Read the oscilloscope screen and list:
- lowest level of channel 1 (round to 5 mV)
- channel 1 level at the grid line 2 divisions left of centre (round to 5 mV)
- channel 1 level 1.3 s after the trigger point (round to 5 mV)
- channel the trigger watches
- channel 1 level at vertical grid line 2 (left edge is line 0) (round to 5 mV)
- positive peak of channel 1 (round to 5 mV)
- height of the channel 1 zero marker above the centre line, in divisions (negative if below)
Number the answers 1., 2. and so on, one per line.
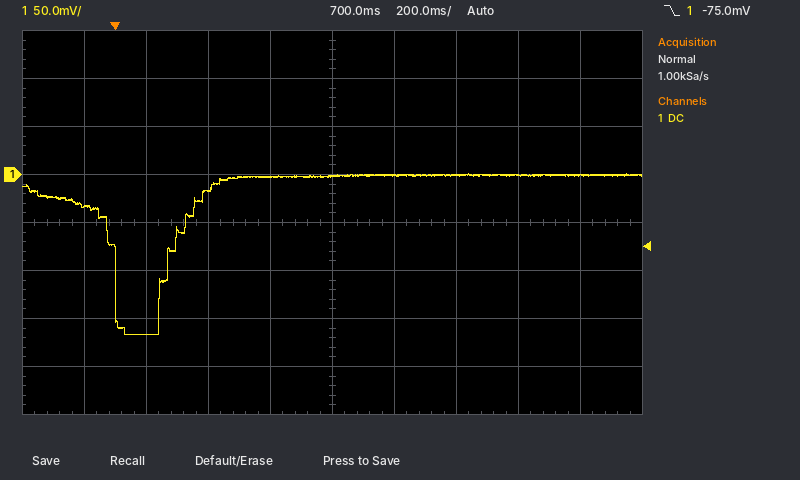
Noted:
1. -165 mV
2. -15 mV
3. 0 mV
4. channel 1
5. -165 mV
6. 0 mV
7. +1.0 div
